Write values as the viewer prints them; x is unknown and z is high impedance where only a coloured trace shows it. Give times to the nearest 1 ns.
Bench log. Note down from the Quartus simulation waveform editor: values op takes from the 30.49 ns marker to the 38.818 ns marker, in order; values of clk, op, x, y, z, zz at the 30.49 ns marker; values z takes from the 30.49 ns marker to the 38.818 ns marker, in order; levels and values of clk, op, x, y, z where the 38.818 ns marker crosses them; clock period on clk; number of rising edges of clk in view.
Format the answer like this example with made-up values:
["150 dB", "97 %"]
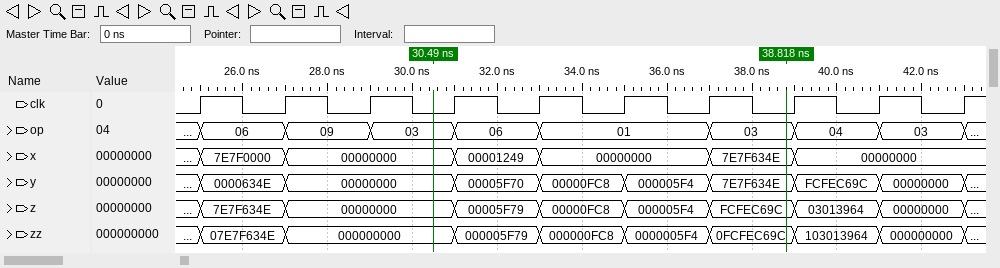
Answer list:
["03, 06, 01, 03", "clk=0, op=03, x=00000000, y=00000000, z=00000000, zz=000000000", "00000000, 00005F79, 00000FC8, 000005F4, FCFEC69C", "clk=0, op=03, x=7E7F634E, y=7E7F634E, z=FCFEC69C", "2 ns", "10"]
